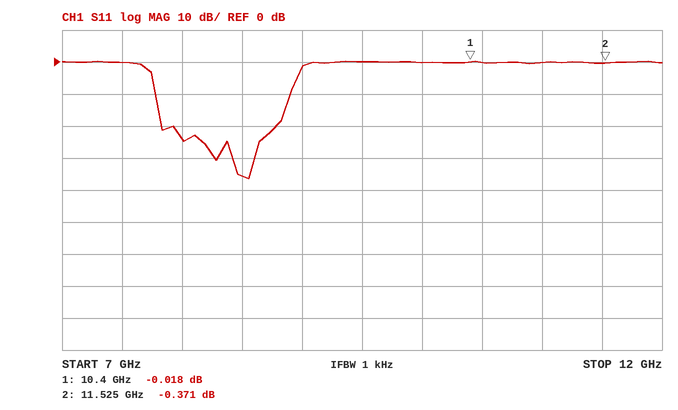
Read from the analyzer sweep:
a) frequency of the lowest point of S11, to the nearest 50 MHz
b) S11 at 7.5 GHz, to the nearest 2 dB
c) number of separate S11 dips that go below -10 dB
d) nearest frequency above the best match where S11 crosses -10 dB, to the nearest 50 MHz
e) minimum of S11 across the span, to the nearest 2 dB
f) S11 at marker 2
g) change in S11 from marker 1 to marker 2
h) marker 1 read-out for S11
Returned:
8.55 GHz
0 dB
2
8.90 GHz
-36 dB
-0.371 dB
-0.353 dB
-0.018 dB
